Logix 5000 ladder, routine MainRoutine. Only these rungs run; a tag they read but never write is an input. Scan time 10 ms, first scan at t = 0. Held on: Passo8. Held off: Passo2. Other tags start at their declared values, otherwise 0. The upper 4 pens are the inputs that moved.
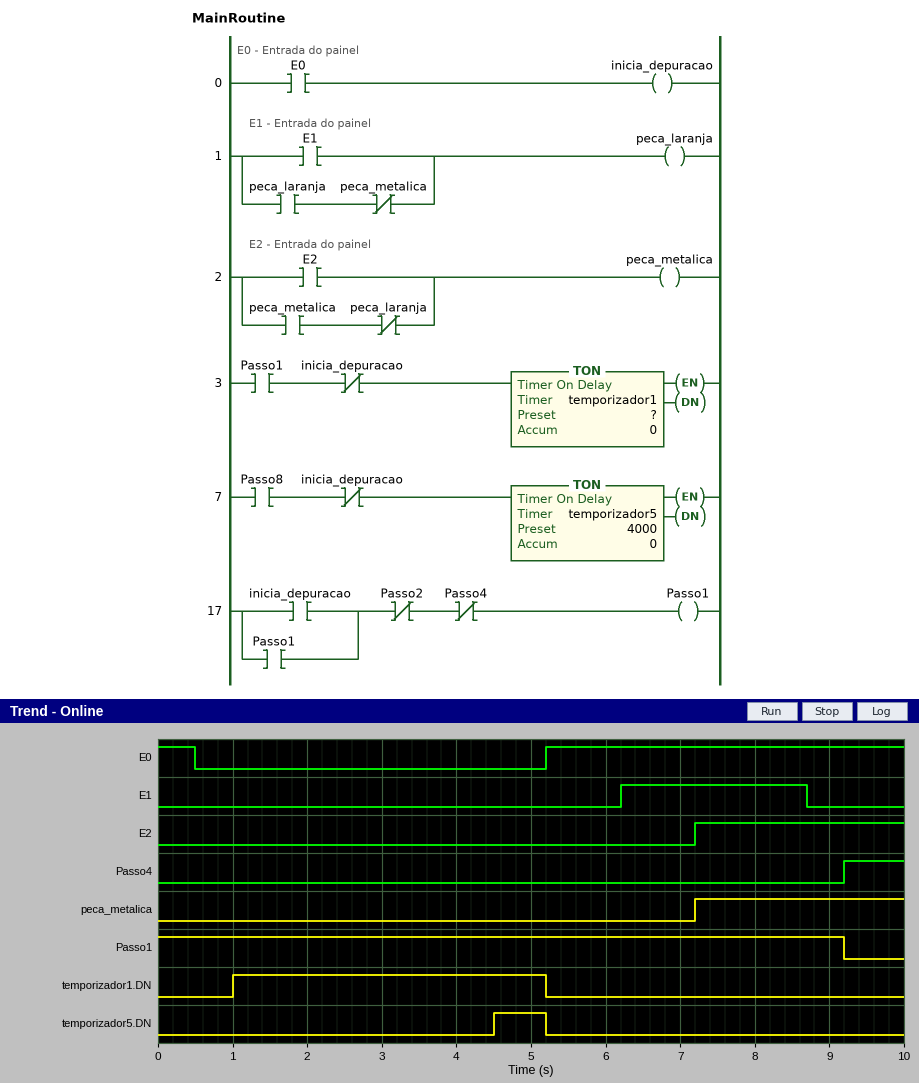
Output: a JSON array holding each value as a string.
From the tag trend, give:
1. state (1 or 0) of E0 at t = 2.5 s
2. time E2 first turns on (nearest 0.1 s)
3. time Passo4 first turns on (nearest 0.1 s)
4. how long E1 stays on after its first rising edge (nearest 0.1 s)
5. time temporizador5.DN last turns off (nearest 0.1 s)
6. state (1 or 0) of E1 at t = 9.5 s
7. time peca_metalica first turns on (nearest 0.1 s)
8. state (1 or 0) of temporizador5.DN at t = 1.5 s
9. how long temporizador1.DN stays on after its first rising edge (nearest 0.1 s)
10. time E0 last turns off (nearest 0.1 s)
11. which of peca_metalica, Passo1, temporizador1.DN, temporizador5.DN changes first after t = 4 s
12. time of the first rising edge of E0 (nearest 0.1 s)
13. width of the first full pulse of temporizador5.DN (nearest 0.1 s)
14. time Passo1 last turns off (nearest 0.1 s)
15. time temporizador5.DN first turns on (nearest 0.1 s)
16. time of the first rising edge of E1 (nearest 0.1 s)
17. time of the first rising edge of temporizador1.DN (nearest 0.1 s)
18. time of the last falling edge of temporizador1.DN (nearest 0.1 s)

["0", "7.2 s", "9.2 s", "2.5 s", "5.2 s", "0", "7.2 s", "0", "4.2 s", "0.5 s", "temporizador5.DN", "5.2 s", "0.7 s", "9.2 s", "4.5 s", "6.2 s", "1.0 s", "5.2 s"]
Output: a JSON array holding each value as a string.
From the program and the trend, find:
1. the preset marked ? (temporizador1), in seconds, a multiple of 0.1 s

["0.5 s"]
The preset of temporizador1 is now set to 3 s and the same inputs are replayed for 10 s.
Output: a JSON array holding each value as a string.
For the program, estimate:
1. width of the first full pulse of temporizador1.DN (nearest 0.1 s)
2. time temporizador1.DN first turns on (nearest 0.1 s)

["1.7 s", "3.5 s"]
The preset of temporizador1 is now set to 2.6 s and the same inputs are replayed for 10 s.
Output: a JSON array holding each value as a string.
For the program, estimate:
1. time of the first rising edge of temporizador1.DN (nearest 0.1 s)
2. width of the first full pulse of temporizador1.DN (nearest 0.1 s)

["3.1 s", "2.1 s"]
